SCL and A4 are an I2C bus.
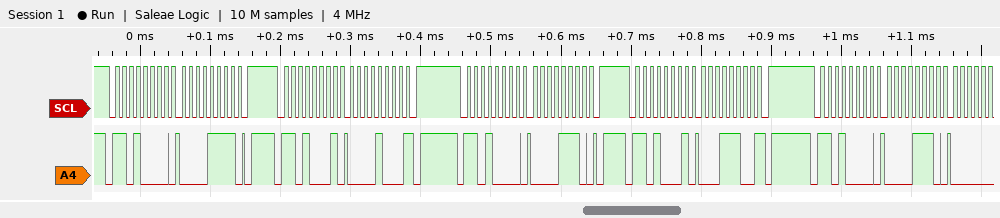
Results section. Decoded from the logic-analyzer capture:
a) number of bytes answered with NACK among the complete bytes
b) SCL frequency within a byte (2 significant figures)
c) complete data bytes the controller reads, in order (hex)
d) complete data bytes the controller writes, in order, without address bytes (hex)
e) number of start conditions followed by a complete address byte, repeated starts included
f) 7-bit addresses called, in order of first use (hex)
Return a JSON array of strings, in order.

["2", "100 kHz", "08 1C", "0F 0E 0E", "5", "0x68"]
